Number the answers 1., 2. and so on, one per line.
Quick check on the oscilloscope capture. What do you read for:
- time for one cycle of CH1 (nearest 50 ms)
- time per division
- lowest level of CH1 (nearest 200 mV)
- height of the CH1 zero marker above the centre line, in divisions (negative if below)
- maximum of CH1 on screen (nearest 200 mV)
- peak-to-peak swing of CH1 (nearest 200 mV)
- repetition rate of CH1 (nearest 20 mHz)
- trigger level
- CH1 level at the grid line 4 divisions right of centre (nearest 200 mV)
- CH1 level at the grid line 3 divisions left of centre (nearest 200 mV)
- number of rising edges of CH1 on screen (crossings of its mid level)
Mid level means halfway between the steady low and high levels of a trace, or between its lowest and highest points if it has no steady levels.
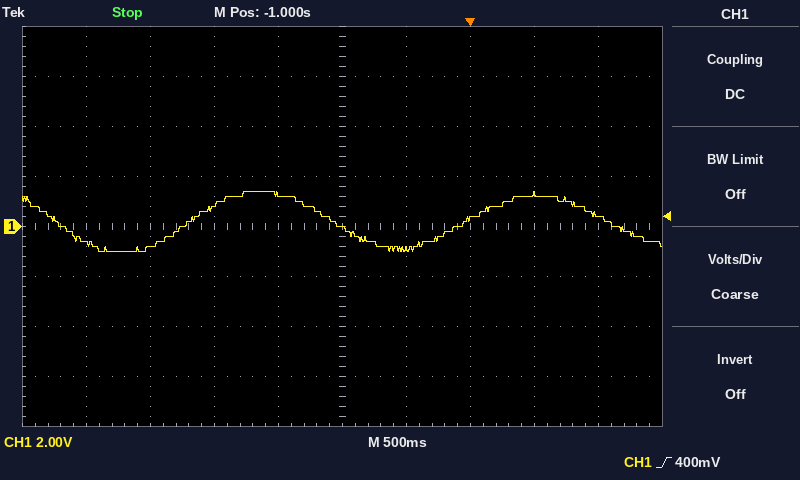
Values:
1. 2.15 s
2. 500 ms
3. -1.0 V
4. 0.0 div
5. 1.4 V
6. 2.4 V
7. 460 mHz
8. 400 mV
9. 400 mV
10. -800 mV
11. 2
